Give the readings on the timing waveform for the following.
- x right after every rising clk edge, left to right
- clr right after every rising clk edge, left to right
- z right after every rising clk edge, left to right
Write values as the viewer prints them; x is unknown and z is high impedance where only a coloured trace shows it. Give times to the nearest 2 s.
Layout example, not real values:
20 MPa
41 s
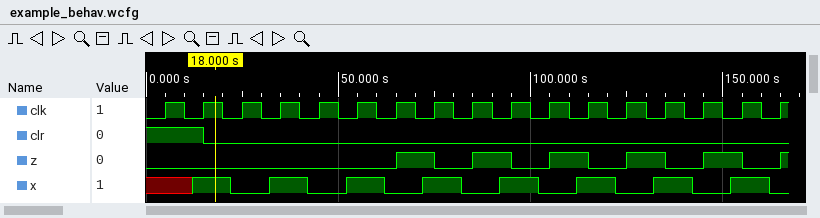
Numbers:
x 1 0 1 0 1 0 1 0 1 0 1 0 1 0 1 0
1 0 0 0 0 0 0 0 0 0 0 0 0 0 0 0 0
0 0 0 0 0 0 1 0 1 0 1 0 1 0 1 0 1
